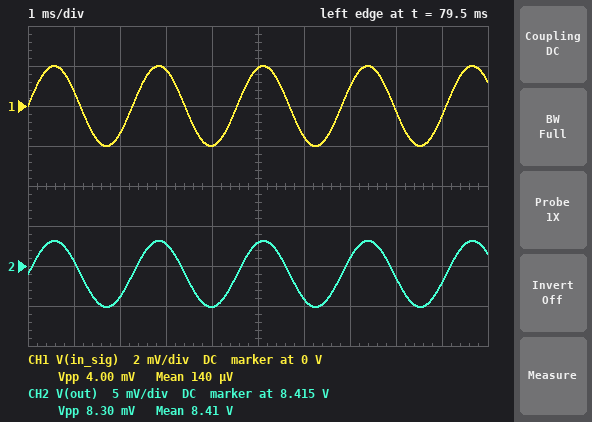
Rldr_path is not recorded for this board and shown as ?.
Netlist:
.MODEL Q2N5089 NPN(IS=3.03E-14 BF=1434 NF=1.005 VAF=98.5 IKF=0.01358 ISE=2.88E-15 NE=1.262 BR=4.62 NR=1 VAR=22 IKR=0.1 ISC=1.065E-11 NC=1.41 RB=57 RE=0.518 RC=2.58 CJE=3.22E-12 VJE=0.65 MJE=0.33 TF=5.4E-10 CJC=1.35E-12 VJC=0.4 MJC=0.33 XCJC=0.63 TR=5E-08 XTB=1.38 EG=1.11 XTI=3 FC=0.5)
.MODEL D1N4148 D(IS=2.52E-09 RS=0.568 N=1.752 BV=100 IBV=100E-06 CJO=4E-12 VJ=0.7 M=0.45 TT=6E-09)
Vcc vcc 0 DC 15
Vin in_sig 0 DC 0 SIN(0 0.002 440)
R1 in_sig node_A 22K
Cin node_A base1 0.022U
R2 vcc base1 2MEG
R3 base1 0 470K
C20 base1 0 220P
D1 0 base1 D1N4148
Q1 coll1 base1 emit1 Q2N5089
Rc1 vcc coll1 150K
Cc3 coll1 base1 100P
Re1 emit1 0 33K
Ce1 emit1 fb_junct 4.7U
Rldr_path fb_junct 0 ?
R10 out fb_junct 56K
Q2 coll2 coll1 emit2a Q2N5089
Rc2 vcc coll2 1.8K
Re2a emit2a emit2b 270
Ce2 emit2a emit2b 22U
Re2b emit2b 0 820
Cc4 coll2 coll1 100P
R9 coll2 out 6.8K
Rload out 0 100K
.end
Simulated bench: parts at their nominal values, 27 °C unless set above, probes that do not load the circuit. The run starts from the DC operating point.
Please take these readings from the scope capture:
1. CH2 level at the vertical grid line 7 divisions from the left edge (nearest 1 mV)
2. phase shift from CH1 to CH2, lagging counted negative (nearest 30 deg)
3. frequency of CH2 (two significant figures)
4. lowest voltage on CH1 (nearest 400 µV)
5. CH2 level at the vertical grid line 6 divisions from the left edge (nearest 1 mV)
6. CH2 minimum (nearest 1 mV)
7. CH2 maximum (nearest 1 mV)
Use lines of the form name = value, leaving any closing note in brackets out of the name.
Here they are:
CH2 level at the vertical grid line 7 divisions from the left edge = 8.416 V
phase shift from CH1 to CH2, lagging counted negative = 0 deg
frequency of CH2 = 440 Hz
lowest voltage on CH1 = -2.0 mV
CH2 level at the vertical grid line 6 divisions from the left edge = 8.411 V
CH2 minimum = 8.410 V
CH2 maximum = 8.418 V
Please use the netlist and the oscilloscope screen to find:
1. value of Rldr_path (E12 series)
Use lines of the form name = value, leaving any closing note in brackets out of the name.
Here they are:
value of Rldr_path = 390 kΩ
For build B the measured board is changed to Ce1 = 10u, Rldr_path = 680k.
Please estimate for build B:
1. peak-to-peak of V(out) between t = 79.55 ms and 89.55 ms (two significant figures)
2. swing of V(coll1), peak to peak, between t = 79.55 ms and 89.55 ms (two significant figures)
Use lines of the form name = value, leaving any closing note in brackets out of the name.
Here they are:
peak-to-peak of V(out) between t = 79.55 ms and 89.55 ms = 8.1 mV
swing of V(coll1), peak to peak, between t = 79.55 ms and 89.55 ms = 4.4 mV
